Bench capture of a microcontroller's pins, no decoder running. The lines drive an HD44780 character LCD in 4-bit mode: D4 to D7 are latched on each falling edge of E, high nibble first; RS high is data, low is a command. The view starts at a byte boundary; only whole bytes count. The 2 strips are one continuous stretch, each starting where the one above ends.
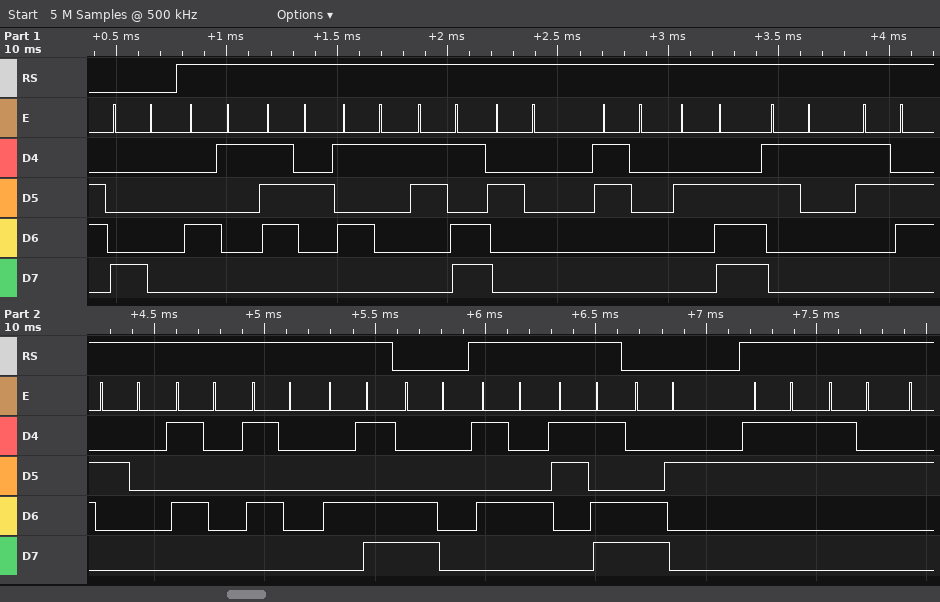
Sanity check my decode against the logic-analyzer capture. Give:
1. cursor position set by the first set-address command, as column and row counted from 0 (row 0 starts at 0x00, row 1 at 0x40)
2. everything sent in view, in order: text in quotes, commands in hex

column 0, row 0
0x80 "ArQ= 0.16 PPM" 0xC0 "T=" 0xC2 "32"
